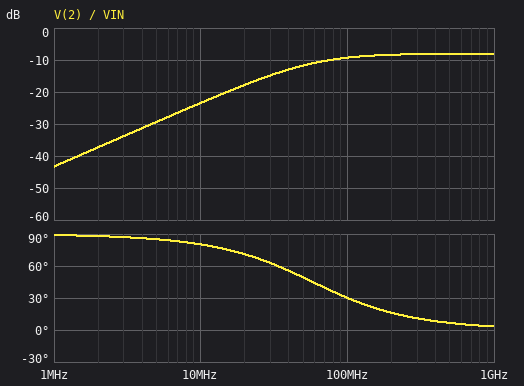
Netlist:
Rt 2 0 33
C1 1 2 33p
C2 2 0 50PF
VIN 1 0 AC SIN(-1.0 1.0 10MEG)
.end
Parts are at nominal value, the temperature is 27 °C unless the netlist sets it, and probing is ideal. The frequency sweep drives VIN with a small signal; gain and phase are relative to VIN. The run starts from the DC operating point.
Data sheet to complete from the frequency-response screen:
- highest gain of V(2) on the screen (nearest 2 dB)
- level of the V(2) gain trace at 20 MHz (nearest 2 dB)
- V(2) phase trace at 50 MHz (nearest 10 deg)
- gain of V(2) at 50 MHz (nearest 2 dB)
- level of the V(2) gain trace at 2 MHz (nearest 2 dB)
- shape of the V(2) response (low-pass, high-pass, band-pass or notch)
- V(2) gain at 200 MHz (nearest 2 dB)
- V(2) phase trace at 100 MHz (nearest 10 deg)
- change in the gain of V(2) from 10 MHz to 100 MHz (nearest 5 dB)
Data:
-8 dB
-18 dB
50 deg
-12 dB
-38 dB
high-pass
-8 dB
30 deg
15 dB
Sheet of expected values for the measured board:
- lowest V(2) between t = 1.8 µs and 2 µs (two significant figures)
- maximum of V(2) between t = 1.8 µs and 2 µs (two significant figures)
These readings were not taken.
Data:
-67 mV
67 mV
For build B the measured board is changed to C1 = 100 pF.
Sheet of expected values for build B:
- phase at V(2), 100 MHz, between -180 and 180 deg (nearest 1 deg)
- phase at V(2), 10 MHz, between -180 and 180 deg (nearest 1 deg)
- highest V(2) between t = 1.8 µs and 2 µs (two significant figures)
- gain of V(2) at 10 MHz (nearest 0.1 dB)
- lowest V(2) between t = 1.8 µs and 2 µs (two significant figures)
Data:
18 deg
73 deg
200 mV
-14.1 dB
-200 mV
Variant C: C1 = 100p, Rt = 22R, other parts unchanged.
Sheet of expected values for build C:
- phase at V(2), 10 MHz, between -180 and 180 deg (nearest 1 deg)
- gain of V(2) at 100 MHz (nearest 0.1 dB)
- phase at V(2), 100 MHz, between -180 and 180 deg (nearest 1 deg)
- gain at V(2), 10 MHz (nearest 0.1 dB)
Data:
78 deg
-4.4 dB
26 deg
-17.4 dB
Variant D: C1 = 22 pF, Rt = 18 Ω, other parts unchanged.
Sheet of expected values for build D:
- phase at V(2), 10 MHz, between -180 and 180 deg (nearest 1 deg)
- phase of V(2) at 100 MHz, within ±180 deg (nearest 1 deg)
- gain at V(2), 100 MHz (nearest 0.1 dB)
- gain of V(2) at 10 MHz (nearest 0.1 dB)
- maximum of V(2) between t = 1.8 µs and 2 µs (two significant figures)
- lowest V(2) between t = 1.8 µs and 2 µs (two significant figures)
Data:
85 deg
51 deg
-14.3 dB
-32.1 dB
25 mV
-25 mV
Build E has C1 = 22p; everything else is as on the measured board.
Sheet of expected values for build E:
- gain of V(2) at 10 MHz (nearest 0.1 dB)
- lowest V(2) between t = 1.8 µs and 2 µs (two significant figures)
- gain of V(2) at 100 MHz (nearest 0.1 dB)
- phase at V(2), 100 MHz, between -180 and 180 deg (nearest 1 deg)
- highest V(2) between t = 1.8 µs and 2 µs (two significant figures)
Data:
-26.9 dB
-45 mV
-11.9 dB
34 deg
45 mV
